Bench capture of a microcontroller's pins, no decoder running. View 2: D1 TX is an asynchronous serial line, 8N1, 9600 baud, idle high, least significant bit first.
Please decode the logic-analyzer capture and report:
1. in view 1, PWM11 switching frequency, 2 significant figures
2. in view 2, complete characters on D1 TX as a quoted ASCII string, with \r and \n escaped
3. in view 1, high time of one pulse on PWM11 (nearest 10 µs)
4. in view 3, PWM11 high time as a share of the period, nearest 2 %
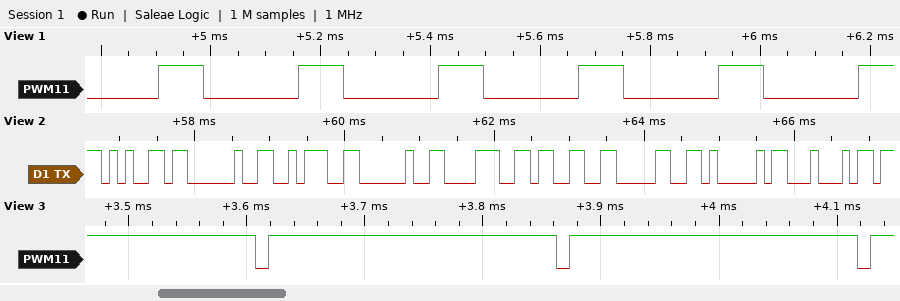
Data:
3.9 kHz
"e : 830AD"
80 µs
96 %
